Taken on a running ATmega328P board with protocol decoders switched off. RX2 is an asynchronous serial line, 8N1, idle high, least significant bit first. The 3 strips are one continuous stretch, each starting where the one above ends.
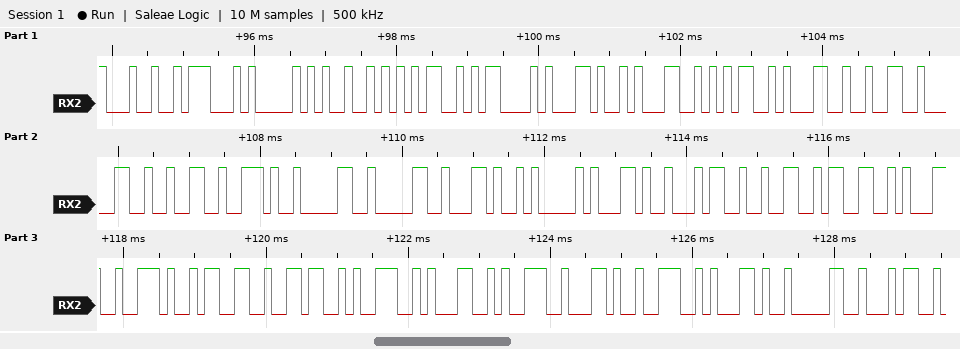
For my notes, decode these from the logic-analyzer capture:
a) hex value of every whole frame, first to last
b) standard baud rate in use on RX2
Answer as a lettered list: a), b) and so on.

a) 24 47 50 52 4D 43 2C 31 35 31 32 30 32 2E 30 30 2C 41 2C 34 32 33 31 2E 33 36 39 31 39 2C 4E 2C 30 34
b) 9600 baud
